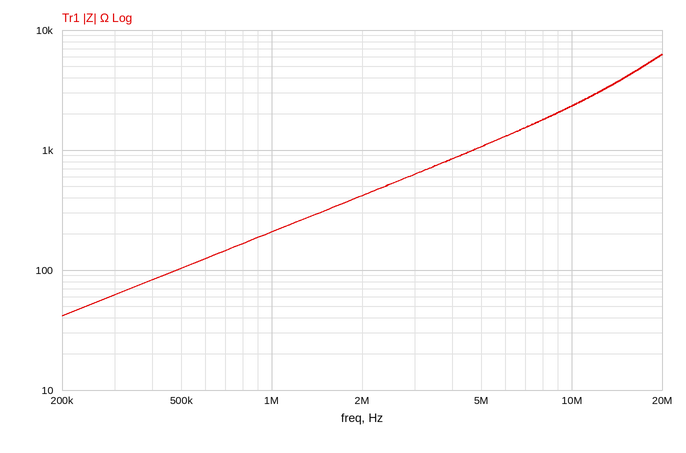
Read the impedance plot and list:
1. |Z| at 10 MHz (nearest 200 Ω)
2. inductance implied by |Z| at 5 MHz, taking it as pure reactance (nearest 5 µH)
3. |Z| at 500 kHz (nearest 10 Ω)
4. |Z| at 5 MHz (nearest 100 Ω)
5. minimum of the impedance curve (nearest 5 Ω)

2.4 kΩ
35 µH
100 Ω
1.1 kΩ
40 Ω
